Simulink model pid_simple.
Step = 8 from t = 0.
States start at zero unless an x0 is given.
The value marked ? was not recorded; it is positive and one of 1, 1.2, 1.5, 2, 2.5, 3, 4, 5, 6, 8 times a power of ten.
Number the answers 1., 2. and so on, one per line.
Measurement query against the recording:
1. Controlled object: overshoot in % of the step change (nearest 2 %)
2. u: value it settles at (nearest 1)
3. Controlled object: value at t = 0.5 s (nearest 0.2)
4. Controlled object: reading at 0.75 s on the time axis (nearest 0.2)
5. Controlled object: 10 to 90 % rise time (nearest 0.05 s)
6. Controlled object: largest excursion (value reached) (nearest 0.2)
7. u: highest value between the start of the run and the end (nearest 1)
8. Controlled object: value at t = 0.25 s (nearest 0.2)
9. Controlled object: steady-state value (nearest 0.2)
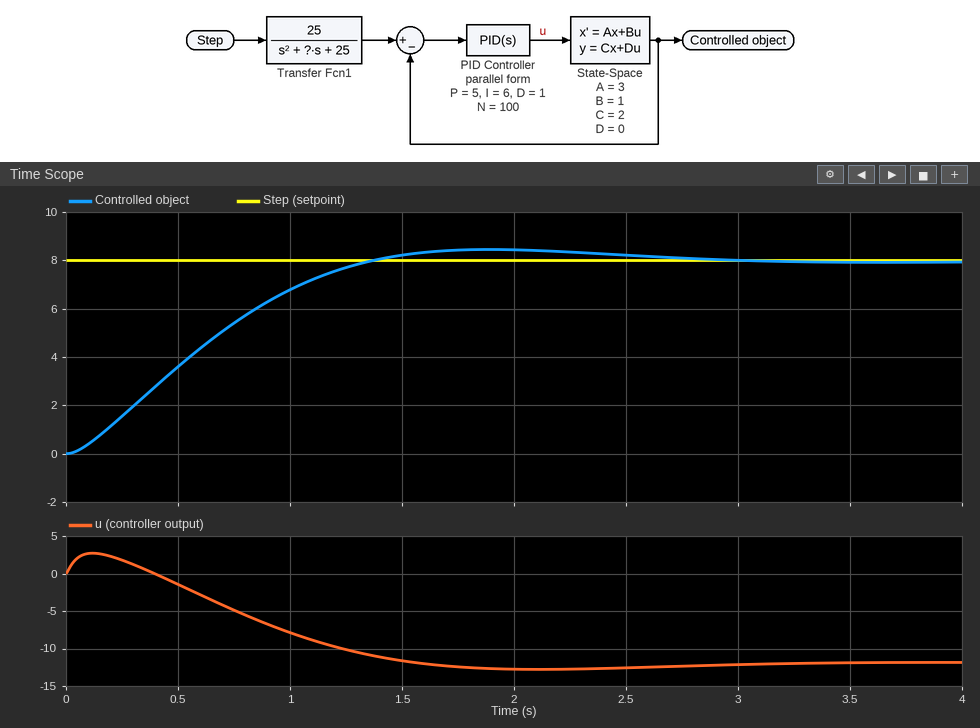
1. 6 %
2. -12
3. 3.6
4. 5.4
5. 0.95 s
6. 8.4
7. 3
8. 1.6
9. 8.0
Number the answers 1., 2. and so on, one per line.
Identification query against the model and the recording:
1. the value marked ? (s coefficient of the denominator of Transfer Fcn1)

1. 20
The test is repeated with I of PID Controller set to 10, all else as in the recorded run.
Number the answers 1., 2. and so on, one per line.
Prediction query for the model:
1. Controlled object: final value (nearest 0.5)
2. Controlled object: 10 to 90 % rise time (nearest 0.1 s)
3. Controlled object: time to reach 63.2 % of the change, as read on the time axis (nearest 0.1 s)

1. 8.0
2. 1.0 s
3. 0.7 s
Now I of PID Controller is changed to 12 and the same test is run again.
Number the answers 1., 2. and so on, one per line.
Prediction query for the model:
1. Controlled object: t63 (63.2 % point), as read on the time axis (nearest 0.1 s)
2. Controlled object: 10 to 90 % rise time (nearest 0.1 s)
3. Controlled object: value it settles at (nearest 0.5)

1. 0.7 s
2. 1.0 s
3. 8.0
